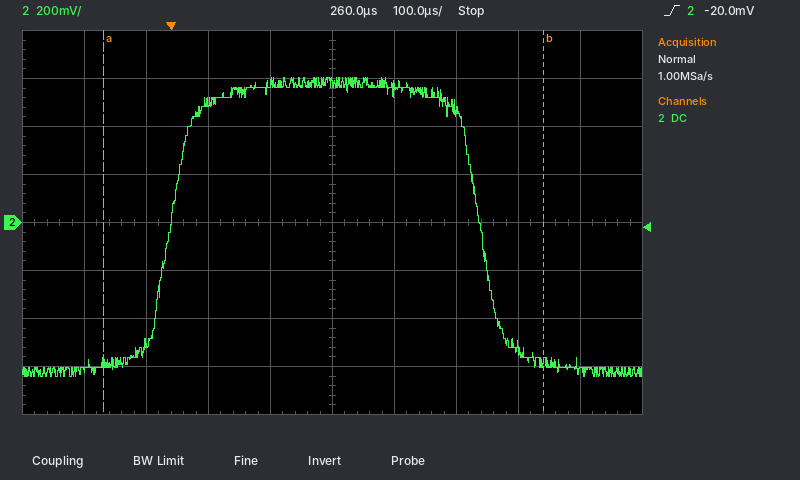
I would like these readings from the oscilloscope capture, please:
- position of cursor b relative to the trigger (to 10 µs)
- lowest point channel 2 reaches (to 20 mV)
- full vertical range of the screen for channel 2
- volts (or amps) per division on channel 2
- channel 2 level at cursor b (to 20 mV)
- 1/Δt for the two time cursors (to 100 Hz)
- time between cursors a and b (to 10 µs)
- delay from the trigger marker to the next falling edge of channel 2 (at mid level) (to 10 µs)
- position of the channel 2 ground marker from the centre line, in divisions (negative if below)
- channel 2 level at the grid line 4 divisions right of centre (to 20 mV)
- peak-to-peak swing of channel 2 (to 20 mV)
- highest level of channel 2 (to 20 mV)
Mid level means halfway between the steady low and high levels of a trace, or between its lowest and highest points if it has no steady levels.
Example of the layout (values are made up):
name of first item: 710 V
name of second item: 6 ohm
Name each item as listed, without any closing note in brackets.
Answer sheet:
position of cursor b relative to the trigger: +600 µs
lowest point channel 2 reaches: -640 mV
full vertical range of the screen for channel 2: 1.6 V
volts (or amps) per division on channel 2: 200 mV
channel 2 level at cursor b: -580 mV
1/Δt for the two time cursors: 1.4 kHz
time between cursors a and b: 710 µs
delay from the trigger marker to the next falling edge of channel 2 (at mid level): 500 µs
position of the channel 2 ground marker from the centre line, in divisions: 0.0 div
channel 2 level at the grid line 4 divisions right of centre: -620 mV
peak-to-peak swing of channel 2: 1.24 V
highest level of channel 2: 600 mV
